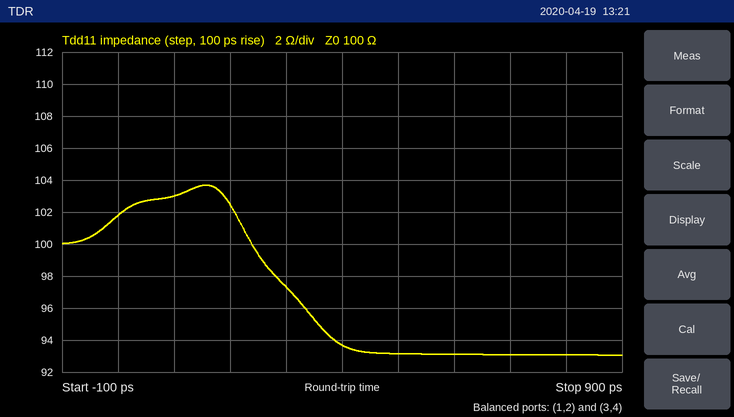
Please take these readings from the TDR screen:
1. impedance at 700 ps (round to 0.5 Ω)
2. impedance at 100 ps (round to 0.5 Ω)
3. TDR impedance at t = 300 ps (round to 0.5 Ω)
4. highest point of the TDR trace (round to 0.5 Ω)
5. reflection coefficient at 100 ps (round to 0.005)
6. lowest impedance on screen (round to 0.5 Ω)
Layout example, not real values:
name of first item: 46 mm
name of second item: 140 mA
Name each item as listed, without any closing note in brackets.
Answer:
impedance at 700 ps: 93.0 Ω
impedance at 100 ps: 103.0 Ω
TDR impedance at t = 300 ps: 97.5 Ω
highest point of the TDR trace: 103.5 Ω
reflection coefficient at 100 ps: +0.015
lowest impedance on screen: 93.0 Ω
